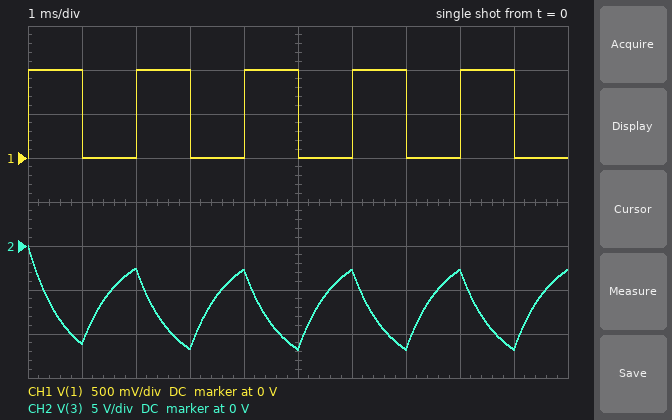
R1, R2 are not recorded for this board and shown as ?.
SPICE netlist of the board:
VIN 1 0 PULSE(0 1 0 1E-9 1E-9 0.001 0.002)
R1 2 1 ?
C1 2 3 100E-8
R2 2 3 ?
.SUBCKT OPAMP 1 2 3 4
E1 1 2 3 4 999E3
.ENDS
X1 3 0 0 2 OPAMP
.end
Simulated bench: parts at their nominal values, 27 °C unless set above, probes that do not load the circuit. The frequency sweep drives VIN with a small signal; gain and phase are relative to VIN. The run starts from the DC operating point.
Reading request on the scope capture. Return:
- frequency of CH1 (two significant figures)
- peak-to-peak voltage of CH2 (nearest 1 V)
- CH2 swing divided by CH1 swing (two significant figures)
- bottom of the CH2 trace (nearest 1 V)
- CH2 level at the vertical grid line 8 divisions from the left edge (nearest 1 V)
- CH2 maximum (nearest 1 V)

500 Hz
12 V
12
-12 V
-3 V
0 V
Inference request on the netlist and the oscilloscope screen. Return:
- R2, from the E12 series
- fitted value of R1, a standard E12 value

680 Ω
47 Ω
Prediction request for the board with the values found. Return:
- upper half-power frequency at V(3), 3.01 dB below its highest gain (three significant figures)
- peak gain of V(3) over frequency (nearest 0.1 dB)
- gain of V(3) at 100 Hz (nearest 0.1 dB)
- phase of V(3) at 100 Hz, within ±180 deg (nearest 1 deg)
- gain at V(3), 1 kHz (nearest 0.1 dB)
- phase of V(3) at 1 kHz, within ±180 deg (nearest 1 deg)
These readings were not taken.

234 Hz
23.2 dB
22.5 dB
157 deg
10.4 dB
103 deg
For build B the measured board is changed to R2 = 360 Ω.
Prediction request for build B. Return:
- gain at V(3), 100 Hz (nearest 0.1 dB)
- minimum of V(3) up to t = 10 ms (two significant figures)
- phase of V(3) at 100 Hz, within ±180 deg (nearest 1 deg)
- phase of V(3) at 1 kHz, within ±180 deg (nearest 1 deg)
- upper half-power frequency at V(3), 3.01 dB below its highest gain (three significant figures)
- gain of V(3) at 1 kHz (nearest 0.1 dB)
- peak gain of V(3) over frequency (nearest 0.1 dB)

17.5 dB
-7.2 V
167 deg
114 deg
442 Hz
9.8 dB
17.7 dB
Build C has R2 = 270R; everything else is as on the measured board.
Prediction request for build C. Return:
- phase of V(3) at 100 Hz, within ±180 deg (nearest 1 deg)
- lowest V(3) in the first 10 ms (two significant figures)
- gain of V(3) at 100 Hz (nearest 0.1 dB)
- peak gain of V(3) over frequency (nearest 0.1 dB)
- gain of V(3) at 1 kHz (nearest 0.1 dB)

170 deg
-5.6 V
15.1 dB
15.2 dB
9.3 dB
